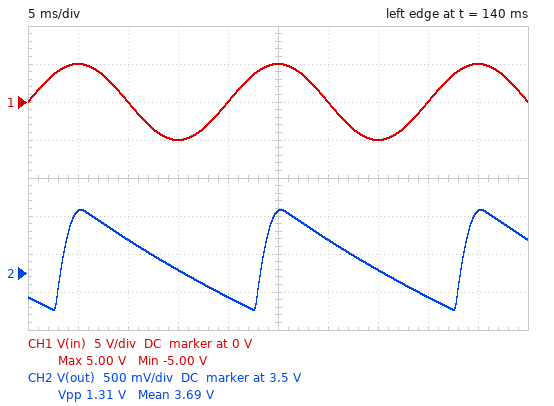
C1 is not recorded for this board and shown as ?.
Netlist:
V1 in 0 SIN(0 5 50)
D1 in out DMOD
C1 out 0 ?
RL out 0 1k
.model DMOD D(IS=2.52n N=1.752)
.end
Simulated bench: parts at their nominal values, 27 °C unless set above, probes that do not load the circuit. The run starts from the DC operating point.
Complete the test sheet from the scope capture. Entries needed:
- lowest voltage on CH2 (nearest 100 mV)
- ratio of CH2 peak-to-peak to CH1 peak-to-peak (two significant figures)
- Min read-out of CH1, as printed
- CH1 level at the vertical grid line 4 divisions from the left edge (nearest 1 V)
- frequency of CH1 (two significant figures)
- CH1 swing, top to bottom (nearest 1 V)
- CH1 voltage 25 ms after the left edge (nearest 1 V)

3.0 V
0.13
-5.00 V
0 V
50 Hz
10 V
5 V
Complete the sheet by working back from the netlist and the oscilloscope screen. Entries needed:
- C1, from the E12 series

47 µF
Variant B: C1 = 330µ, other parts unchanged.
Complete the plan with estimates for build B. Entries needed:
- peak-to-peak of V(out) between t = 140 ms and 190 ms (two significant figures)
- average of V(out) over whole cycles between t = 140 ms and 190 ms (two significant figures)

230 mV
4.2 V
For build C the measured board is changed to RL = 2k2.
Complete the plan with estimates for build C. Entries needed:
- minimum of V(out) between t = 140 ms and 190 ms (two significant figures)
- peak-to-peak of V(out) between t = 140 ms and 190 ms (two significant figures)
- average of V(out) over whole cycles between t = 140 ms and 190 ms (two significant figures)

3.7 V
680 mV
4.0 V
